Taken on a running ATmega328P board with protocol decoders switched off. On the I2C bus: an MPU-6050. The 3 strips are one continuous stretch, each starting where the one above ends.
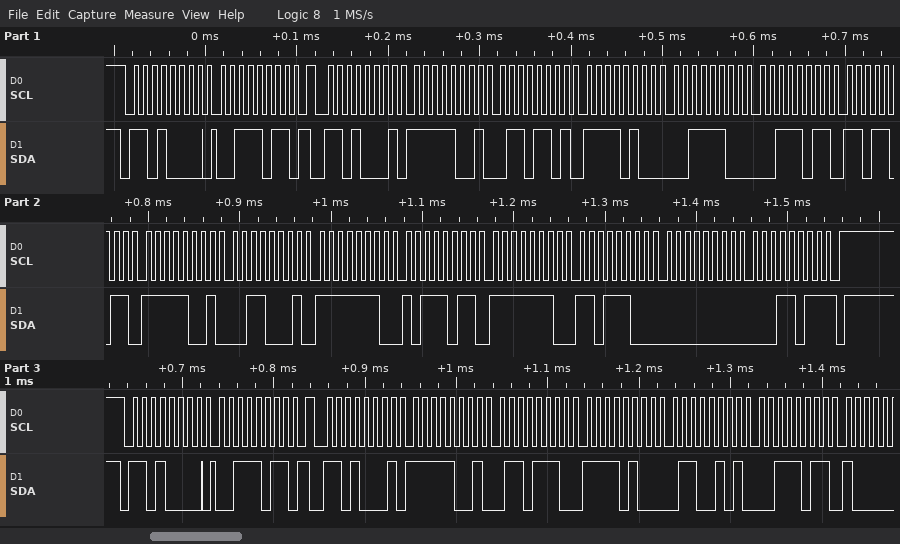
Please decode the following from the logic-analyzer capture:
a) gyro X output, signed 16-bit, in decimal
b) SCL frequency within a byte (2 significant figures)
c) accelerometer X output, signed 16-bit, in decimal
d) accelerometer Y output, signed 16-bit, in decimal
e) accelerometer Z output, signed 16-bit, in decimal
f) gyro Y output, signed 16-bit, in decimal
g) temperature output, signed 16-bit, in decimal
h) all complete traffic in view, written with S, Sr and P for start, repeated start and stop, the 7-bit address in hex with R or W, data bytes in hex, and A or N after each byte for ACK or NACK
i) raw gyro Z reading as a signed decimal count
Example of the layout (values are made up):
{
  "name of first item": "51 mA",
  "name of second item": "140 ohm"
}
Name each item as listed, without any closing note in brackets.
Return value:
{
  "gyro X output, signed 16-bit, in decimal": "-325",
  "SCL frequency within a byte": "100 kHz",
  "accelerometer X output, signed 16-bit, in decimal": "-1683",
  "accelerometer Y output, signed 16-bit, in decimal": "-3012",
  "accelerometer Z output, signed 16-bit, in decimal": "15323",
  "gyro Y output, signed 16-bit, in decimal": "-292",
  "temperature output, signed 16-bit, in decimal": "-1743",
  "all complete traffic in view, written with S, Sr and P for start, repeated start and stop, the 7-bit address in hex with R or W, data bytes in hex, and A or N after each byte for ACK or NACK": "S 68W A 3B A Sr 68R A F9 A 6D A F4 A 3C A 3B A DB A F9 A 31 A FE A BB A FE A DC A 00 A 1B N P S 68W A 3B A Sr 68R A F9 A 6E A F4 A 65 A 3B A",
  "raw gyro Z reading as a signed decimal count": "27"
}
